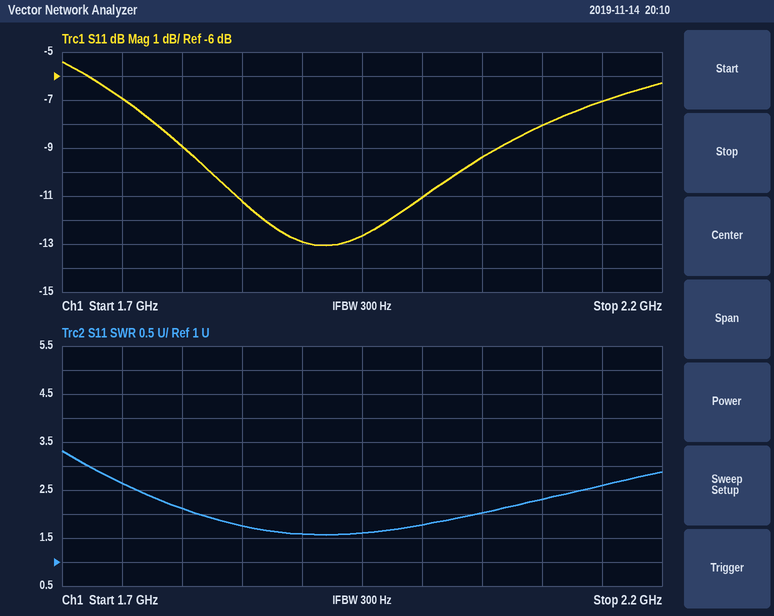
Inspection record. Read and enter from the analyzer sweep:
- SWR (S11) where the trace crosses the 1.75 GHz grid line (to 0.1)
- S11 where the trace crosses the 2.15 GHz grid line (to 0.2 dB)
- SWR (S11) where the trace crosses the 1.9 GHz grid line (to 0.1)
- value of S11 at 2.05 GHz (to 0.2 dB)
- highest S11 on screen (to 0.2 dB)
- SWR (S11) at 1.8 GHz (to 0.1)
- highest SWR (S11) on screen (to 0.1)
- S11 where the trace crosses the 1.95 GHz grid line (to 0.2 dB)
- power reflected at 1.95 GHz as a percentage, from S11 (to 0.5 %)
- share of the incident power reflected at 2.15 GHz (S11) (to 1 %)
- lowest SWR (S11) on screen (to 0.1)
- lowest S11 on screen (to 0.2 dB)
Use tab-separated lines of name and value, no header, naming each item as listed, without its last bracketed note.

SWR (S11) where the trace crosses the 1.75 GHz grid line	2.6
S11 where the trace crosses the 2.15 GHz grid line	-7.0 dB
SWR (S11) where the trace crosses the 1.9 GHz grid line	1.6
value of S11 at 2.05 GHz	-9.4 dB
highest S11 on screen	-5.4 dB
SWR (S11) at 1.8 GHz	2.1
highest SWR (S11) on screen	3.3
S11 where the trace crosses the 1.95 GHz grid line	-12.6 dB
power reflected at 1.95 GHz as a percentage, from S11	5.5 %
share of the incident power reflected at 2.15 GHz (S11)	20 %
lowest SWR (S11) on screen	1.6
lowest S11 on screen	-13.0 dB
